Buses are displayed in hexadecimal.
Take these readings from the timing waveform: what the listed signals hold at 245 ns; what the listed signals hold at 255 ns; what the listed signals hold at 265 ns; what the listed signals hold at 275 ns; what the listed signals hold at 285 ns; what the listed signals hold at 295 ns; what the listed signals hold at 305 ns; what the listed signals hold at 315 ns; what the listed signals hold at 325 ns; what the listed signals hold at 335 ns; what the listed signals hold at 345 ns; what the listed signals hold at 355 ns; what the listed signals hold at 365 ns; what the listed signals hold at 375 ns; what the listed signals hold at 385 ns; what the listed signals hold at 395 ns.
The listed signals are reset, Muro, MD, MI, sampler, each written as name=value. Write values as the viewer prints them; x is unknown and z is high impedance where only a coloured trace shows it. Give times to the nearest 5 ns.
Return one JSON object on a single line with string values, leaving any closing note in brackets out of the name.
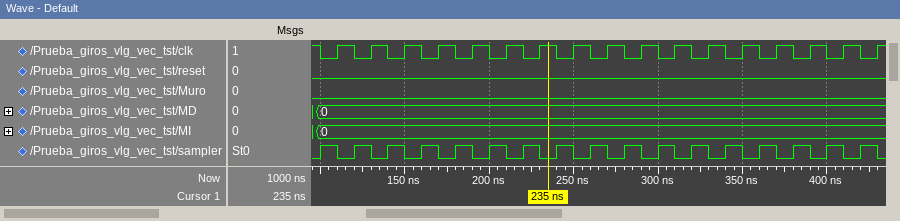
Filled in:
{"what the listed signals hold at 245 ns": "reset=0, Muro=0, MD=0, MI=0, sampler=1", "what the listed signals hold at 255 ns": "reset=0, Muro=0, MD=0, MI=0, sampler=0", "what the listed signals hold at 265 ns": "reset=0, Muro=0, MD=0, MI=0, sampler=1", "what the listed signals hold at 275 ns": "reset=0, Muro=0, MD=0, MI=0, sampler=0", "what the listed signals hold at 285 ns": "reset=0, Muro=0, MD=0, MI=0, sampler=1", "what the listed signals hold at 295 ns": "reset=0, Muro=0, MD=0, MI=0, sampler=0", "what the listed signals hold at 305 ns": "reset=0, Muro=0, MD=0, MI=0, sampler=1", "what the listed signals hold at 315 ns": "reset=0, Muro=0, MD=0, MI=0, sampler=0", "what the listed signals hold at 325 ns": "reset=0, Muro=0, MD=0, MI=0, sampler=1", "what the listed signals hold at 335 ns": "reset=0, Muro=0, MD=0, MI=0, sampler=0", "what the listed signals hold at 345 ns": "reset=0, Muro=0, MD=0, MI=0, sampler=1", "what the listed signals hold at 355 ns": "reset=0, Muro=0, MD=0, MI=0, sampler=0", "what the listed signals hold at 365 ns": "reset=0, Muro=0, MD=0, MI=0, sampler=1", "what the listed signals hold at 375 ns": "reset=0, Muro=0, MD=0, MI=0, sampler=0", "what the listed signals hold at 385 ns": "reset=0, Muro=0, MD=0, MI=0, sampler=1", "what the listed signals hold at 395 ns": "reset=0, Muro=0, MD=0, MI=0, sampler=0"}
